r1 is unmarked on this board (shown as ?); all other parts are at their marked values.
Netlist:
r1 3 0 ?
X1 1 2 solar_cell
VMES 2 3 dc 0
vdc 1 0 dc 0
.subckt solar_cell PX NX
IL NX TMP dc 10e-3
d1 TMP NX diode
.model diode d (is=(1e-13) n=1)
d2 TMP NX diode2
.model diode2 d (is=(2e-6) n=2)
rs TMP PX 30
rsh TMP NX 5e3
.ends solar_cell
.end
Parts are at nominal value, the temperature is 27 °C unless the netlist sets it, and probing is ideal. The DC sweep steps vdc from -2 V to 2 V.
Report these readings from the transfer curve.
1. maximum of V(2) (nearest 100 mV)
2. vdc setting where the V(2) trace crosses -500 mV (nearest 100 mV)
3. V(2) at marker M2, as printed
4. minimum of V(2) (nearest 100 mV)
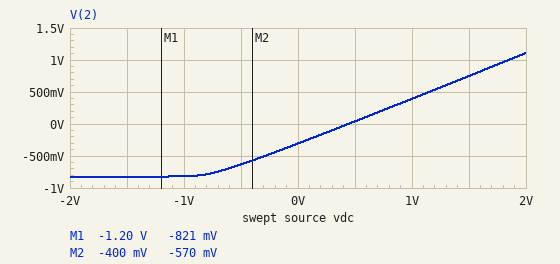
1.1 V
-300 mV
-570 mV
-800 mV
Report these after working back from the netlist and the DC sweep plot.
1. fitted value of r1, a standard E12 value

82 Ω
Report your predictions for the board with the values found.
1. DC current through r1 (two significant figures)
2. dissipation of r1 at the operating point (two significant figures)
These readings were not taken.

3.7 mA
1.1 mW
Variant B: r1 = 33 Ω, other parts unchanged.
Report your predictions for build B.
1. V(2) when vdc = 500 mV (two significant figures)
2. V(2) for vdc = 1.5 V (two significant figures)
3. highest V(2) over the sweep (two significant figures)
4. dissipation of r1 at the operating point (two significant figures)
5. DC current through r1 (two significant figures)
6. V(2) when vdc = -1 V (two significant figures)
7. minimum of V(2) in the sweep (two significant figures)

29 mV
530 mV
780 mV
1.3 mW
6.2 mA
-330 mV
-340 mV
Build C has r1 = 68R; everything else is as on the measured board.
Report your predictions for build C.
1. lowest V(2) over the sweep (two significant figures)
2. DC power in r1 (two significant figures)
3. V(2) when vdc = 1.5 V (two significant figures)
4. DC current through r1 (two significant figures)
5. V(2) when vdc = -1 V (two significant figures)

-690 mV
1.2 mW
710 mV
4.2 mA
-680 mV
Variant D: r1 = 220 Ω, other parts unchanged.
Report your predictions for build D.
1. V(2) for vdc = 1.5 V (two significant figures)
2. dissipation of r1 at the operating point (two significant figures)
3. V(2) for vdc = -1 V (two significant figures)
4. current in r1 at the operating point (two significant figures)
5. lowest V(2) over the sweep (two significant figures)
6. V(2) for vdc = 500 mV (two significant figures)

920 mV
650 µW
-1.2 V
1.7 mA
-2.0 V
52 mV
